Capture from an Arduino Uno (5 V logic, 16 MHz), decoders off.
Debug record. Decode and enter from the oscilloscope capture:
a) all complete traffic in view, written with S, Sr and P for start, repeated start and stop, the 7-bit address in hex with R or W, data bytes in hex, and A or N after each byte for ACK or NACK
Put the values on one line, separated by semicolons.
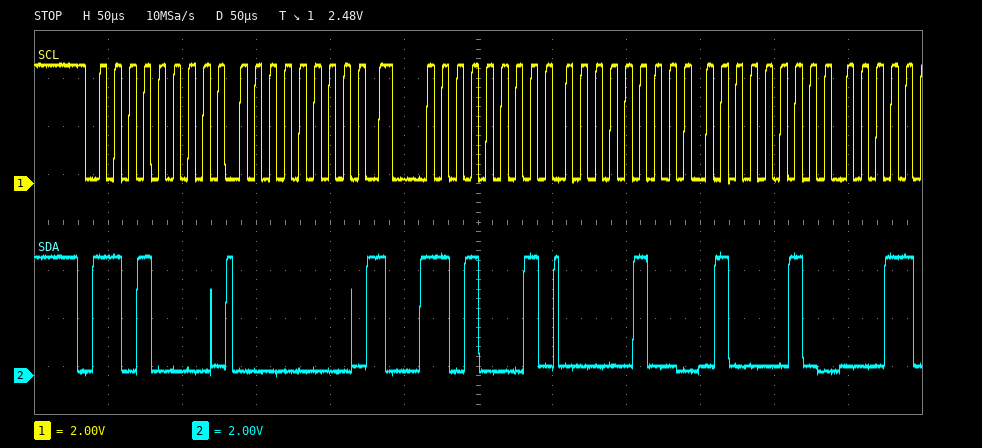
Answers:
S 68W A 00 A Sr 68R A 04 A 42 A
